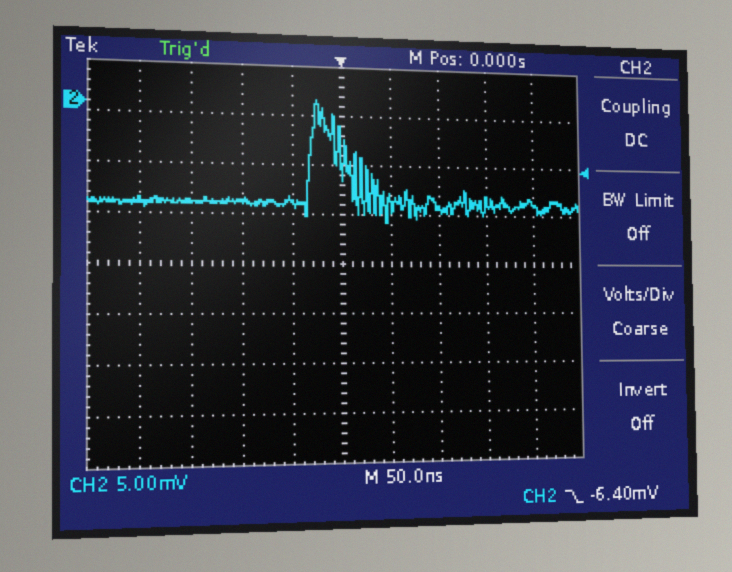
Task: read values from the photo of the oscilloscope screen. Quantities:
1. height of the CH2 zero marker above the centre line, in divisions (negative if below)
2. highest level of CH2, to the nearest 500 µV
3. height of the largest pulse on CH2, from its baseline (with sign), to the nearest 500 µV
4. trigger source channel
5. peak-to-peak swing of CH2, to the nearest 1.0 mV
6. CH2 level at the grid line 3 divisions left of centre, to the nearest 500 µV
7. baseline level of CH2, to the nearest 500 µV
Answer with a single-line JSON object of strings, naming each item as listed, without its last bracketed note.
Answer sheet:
{"height of the CH2 zero marker above the centre line, in divisions": "+3.2 div", "highest level of CH2, to the nearest 500 µV": "500 µV", "height of the largest pulse on CH2, from its baseline (with sign), to the nearest 500 µV": "+10.5 mV", "trigger source channel": "CH2", "peak-to-peak swing of CH2, to the nearest 1.0 mV": "12.0 mV", "CH2 level at the grid line 3 divisions left of centre, to the nearest 500 µV": "-10.0 mV", "baseline level of CH2, to the nearest 500 µV": "-10.0 mV"}
